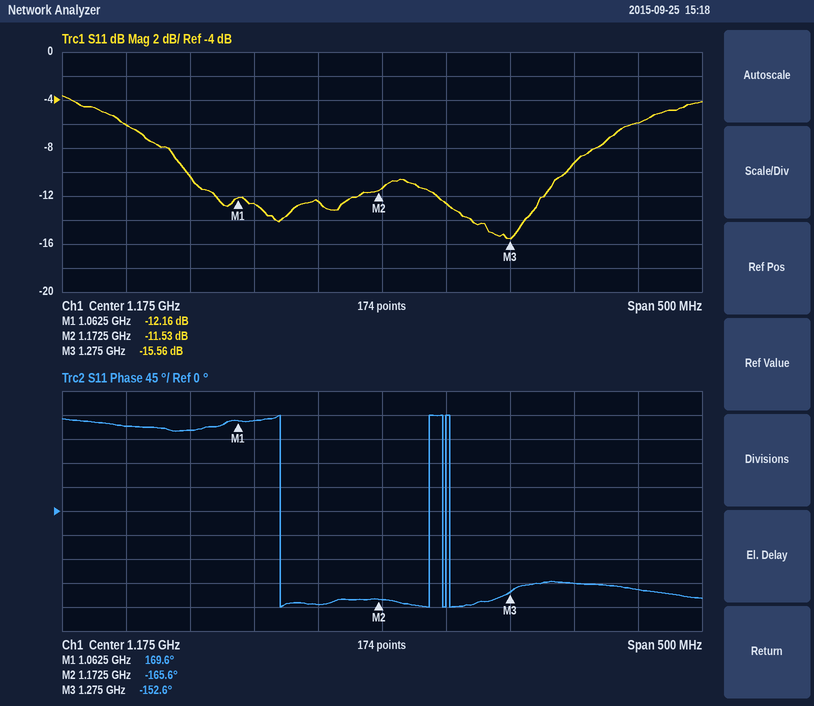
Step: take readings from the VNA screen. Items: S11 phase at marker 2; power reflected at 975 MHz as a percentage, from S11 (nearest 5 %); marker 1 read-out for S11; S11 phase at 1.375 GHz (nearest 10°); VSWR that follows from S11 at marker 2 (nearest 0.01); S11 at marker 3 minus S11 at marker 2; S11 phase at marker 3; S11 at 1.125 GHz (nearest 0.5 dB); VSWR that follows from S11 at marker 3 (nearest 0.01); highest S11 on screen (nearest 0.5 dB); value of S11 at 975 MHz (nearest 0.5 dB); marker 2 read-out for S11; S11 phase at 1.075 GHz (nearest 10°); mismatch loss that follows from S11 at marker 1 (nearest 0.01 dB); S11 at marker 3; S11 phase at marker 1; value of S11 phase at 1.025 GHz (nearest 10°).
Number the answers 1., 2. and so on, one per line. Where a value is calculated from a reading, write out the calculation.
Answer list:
1. -165.6°
2. 10^(-6/10) ≈ 25 %
3. -12.16 dB
4. -150°
5. (1 + 0.2652)/(1 − 0.2652) ≈ 1.72
6. -15.56 − (-11.53) = -4.03 dB
7. -152.6°
8. -12.5 dB
9. (1 + 0.1667)/(1 − 0.1667) ≈ 1.40
10. -3.5 dB
11. -6.0 dB
12. -11.53 dB
13. 170°
14. −10 log10(1 − 10^(-12.16/10)) ≈ 0.27 dB
15. -15.56 dB
16. 169.6°
17. 150°
